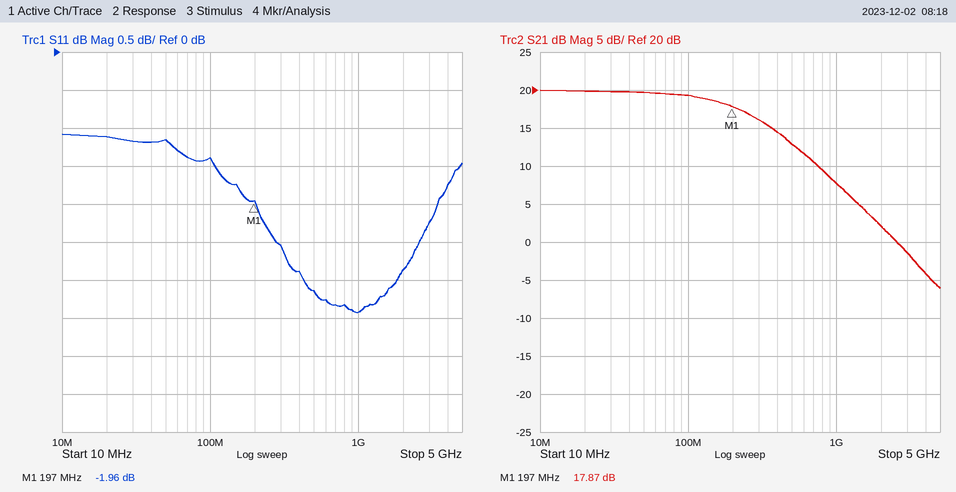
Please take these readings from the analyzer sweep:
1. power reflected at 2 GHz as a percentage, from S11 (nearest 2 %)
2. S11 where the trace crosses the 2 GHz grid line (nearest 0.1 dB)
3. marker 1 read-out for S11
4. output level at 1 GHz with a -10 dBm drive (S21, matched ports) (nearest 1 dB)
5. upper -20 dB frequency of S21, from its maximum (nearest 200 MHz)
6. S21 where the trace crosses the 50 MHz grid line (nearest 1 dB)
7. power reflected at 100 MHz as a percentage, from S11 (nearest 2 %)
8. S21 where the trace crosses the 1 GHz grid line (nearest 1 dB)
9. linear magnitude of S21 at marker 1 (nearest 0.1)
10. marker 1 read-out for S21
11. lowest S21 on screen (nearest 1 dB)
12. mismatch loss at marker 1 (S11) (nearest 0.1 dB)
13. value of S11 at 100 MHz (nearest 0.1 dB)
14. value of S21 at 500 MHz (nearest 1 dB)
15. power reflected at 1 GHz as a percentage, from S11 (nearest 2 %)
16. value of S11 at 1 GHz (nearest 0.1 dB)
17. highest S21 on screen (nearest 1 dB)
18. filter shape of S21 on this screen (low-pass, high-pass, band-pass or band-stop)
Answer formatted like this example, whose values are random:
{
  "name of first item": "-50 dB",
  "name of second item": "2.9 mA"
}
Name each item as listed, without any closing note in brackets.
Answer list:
{
  "power reflected at 2 GHz as a percentage, from S11": "52 %",
  "S11 where the trace crosses the 2 GHz grid line": "-2.9 dB",
  "marker 1 read-out for S11": "-1.96 dB",
  "output level at 1 GHz with a -10 dBm drive (S21, matched ports)": "-2 dBm",
  "upper -20 dB frequency of S21, from its maximum": "2.6 GHz",
  "S21 where the trace crosses the 50 MHz grid line": "20 dB",
  "power reflected at 100 MHz as a percentage, from S11": "72 %",
  "S21 where the trace crosses the 1 GHz grid line": "8 dB",
  "linear magnitude of S21 at marker 1": "7.8",
  "marker 1 read-out for S21": "17.87 dB",
  "lowest S21 on screen": "-6 dB",
  "mismatch loss at marker 1 (S11)": "4.4 dB",
  "value of S11 at 100 MHz": "-1.4 dB",
  "value of S21 at 500 MHz": "13 dB",
  "power reflected at 1 GHz as a percentage, from S11": "46 %",
  "value of S11 at 1 GHz": "-3.4 dB",
  "highest S21 on screen": "20 dB",
  "filter shape of S21 on this screen": "low-pass"
}
